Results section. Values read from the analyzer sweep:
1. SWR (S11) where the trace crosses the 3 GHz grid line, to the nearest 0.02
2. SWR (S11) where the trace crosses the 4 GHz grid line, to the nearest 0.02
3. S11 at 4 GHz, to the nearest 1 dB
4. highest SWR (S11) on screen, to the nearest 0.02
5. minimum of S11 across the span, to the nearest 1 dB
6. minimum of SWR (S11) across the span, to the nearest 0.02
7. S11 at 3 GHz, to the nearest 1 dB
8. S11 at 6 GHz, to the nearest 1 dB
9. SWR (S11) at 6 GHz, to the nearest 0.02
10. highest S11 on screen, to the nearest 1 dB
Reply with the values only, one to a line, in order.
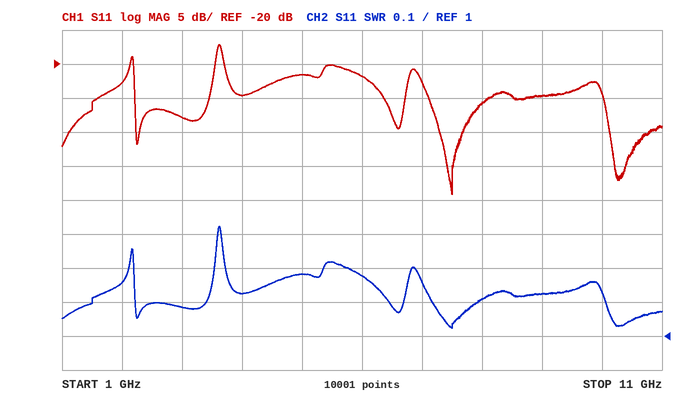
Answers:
1.08
1.12
-25 dB
1.32
-39 dB
1.02
-28 dB
-22 dB
1.18
-17 dB
